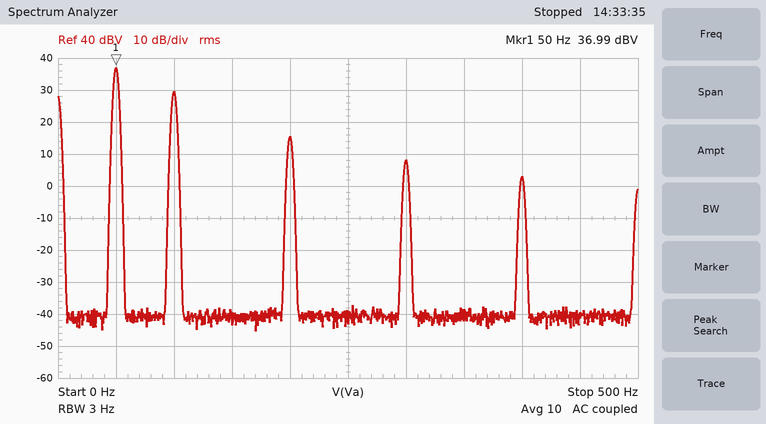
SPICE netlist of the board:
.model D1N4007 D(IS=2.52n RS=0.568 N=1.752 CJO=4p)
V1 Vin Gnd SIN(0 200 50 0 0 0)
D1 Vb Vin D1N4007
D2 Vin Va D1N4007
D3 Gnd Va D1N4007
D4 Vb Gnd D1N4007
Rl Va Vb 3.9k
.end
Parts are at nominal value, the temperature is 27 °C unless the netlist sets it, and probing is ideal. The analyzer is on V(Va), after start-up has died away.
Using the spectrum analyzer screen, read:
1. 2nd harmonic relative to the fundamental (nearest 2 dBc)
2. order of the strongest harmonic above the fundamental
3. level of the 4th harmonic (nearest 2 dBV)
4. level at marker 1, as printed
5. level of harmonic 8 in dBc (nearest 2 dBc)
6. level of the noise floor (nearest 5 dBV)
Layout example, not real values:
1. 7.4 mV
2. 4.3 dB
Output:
1. -8 dBc
2. 2
3. 16 dBV
4. 36.99 dBV
5. -34 dBc
6. -40 dBV
